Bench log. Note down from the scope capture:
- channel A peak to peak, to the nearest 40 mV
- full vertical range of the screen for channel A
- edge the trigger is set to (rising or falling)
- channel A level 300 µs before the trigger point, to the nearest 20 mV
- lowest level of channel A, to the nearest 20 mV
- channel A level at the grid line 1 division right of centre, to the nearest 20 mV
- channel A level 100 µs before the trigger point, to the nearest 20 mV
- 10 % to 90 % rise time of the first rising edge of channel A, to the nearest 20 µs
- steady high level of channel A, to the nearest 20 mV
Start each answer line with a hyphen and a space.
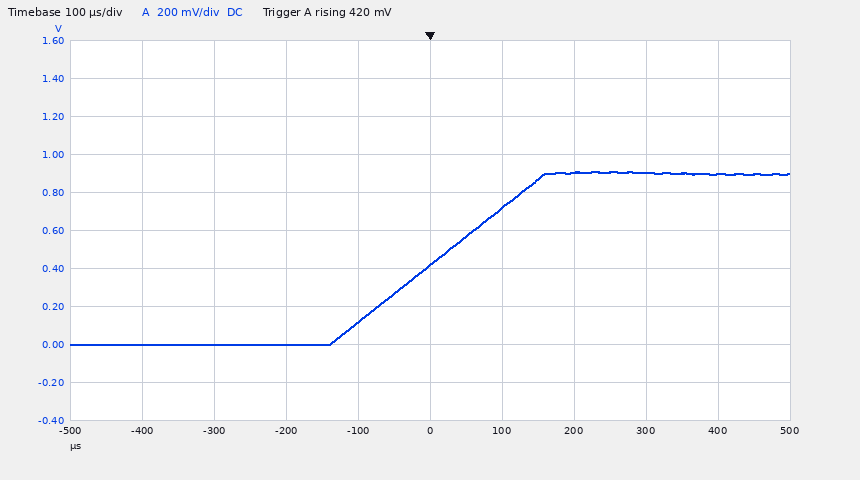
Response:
- 920 mV
- 2 V
- rising
- 0 mV
- 0 mV
- 720 mV
- 120 mV
- 240 µs
- 900 mV
